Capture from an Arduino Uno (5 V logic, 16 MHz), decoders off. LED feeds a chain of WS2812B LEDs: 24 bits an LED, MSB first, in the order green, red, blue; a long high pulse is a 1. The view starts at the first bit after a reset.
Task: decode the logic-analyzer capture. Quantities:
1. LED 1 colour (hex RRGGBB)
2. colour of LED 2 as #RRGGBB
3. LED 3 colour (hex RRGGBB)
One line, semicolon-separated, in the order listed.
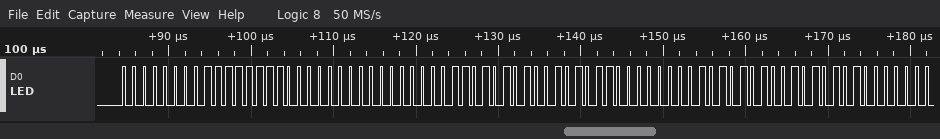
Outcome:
#FF0000; #D5002B; #AA0055
